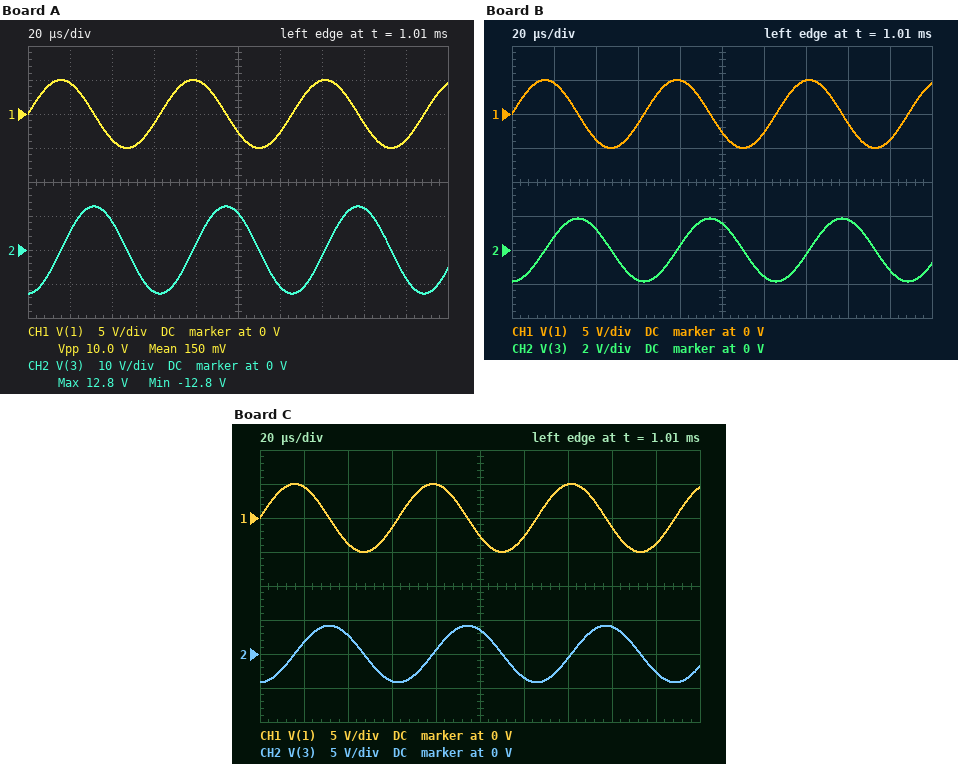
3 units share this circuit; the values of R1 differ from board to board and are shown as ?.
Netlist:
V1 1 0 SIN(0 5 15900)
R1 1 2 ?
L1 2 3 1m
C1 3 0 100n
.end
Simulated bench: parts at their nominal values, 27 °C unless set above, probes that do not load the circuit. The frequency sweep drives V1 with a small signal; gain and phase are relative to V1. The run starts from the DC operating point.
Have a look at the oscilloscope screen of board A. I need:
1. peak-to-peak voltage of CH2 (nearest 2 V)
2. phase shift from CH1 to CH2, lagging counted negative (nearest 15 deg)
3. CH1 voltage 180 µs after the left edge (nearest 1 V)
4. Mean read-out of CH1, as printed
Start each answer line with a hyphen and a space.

- 26 V
- -90 deg
- -4 V
- 150 mV
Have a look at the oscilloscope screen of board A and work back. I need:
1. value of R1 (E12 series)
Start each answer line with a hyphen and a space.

- 39 Ω
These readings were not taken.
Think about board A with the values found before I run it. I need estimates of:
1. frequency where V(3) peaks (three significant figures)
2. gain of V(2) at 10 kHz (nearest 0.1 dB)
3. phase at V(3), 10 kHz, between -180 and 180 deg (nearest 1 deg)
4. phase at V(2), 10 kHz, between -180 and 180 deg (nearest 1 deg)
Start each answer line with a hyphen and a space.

- 15.3 kHz
- -0.7 dB
- -22 deg
- -22 deg
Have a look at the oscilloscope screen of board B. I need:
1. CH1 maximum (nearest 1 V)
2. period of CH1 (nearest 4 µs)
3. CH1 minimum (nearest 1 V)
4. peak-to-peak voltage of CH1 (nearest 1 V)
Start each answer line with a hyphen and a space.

- 5 V
- 64 µs
- -5 V
- 10 V
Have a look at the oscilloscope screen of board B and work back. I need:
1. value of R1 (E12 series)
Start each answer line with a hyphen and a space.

- 270 Ω
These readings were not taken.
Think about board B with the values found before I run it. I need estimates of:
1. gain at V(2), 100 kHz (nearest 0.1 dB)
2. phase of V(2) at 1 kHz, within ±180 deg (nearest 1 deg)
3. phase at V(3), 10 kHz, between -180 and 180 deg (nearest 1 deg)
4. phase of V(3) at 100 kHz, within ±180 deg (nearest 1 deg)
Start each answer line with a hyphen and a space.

- -0.8 dB
- -10 deg
- -70 deg
- -156 deg
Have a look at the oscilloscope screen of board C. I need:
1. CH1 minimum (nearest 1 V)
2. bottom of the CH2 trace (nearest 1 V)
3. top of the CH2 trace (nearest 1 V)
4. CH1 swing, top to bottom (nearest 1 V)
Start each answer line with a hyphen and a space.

- -5 V
- -4 V
- 4 V
- 10 V
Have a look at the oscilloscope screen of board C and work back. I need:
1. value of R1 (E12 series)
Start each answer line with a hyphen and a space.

- 120 Ω
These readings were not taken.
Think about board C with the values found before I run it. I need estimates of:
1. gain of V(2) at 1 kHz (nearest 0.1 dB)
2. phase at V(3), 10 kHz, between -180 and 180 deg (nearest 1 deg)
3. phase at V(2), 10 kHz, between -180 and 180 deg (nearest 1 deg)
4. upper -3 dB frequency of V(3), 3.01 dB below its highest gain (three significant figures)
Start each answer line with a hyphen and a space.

- 0 dB
- -51 deg
- -51 deg
- 17.7 kHz
